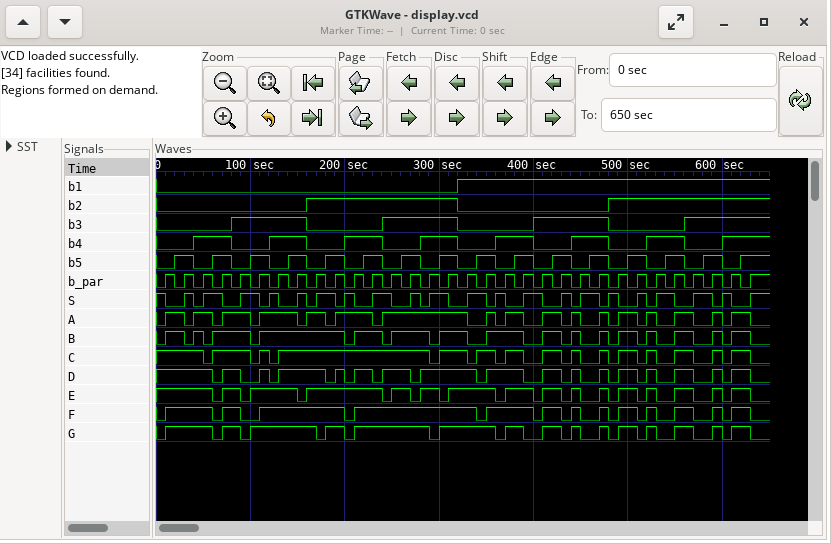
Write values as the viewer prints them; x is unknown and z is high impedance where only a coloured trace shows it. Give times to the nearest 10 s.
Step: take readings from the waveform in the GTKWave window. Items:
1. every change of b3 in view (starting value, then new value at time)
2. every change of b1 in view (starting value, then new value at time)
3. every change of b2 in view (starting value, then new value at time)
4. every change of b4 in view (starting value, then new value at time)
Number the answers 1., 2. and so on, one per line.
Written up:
1. 0, 1 at 80 s, 0 at 160 s, 1 at 240 s, 0 at 320 s, 1 at 400 s, 0 at 480 s, 1 at 560 s
2. 0, 1 at 320 s
3. 0, 1 at 160 s, 0 at 320 s, 1 at 480 s
4. 0, 1 at 40 s, 0 at 80 s, 1 at 120 s, 0 at 160 s, 1 at 200 s, 0 at 240 s, 1 at 280 s, 0 at 320 s, 1 at 360 s, 0 at 400 s, 1 at 440 s, 0 at 480 s, 1 at 520 s, 0 at 560 s, 1 at 600 s
